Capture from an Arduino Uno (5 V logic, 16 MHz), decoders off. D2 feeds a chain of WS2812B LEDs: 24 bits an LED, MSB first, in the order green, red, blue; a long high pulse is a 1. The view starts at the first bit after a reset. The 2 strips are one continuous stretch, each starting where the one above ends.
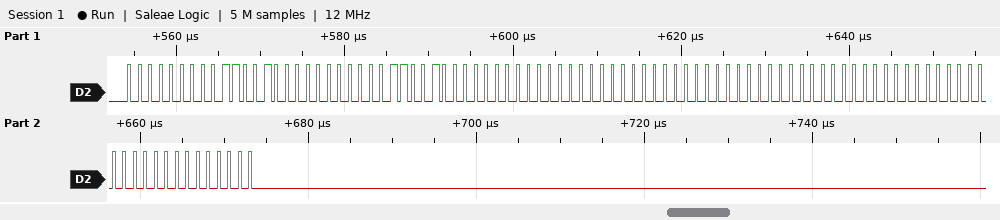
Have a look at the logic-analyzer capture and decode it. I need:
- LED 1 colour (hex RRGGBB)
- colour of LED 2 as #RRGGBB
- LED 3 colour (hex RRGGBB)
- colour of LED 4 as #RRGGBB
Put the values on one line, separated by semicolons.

#640000; #006400; #000000; #000000
